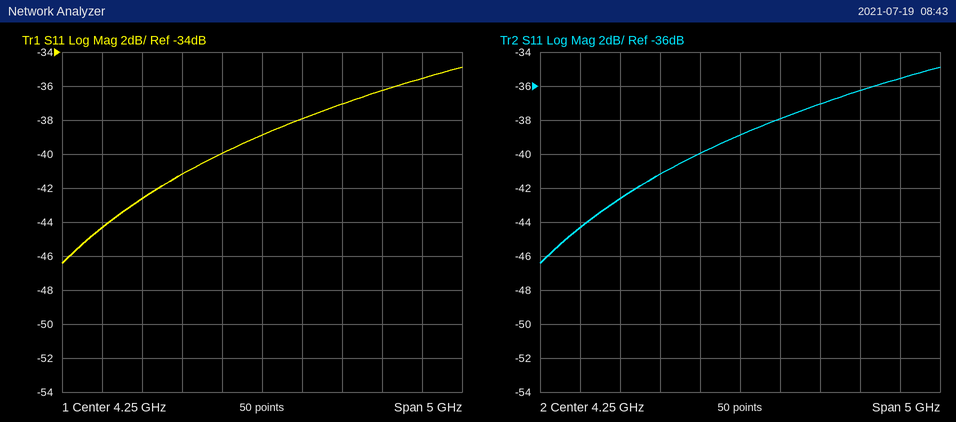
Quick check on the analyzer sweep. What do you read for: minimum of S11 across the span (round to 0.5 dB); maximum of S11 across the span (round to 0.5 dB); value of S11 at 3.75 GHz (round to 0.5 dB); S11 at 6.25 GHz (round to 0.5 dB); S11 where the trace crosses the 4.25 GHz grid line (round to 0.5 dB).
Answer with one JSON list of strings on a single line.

["-46.5 dB", "-35.0 dB", "-40.0 dB", "-35.5 dB", "-39.0 dB"]
